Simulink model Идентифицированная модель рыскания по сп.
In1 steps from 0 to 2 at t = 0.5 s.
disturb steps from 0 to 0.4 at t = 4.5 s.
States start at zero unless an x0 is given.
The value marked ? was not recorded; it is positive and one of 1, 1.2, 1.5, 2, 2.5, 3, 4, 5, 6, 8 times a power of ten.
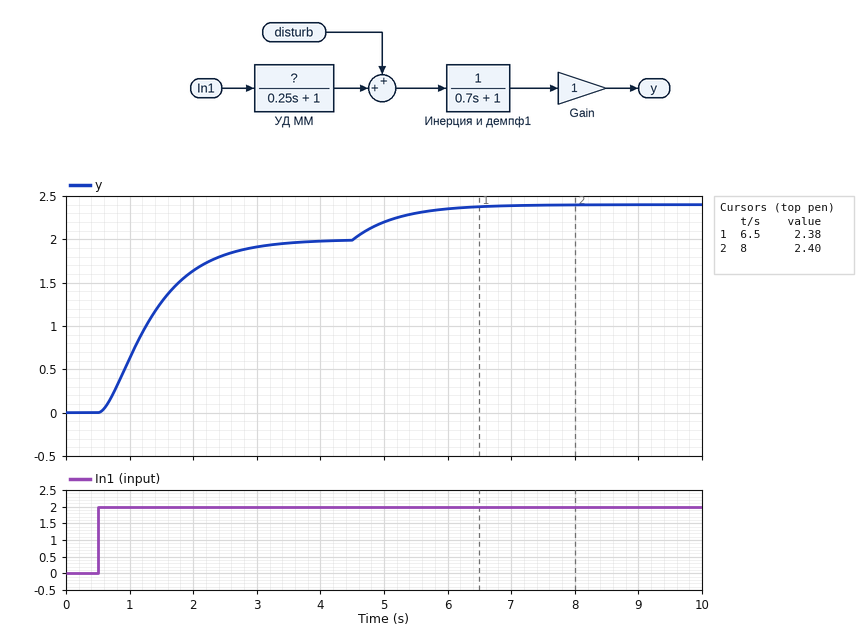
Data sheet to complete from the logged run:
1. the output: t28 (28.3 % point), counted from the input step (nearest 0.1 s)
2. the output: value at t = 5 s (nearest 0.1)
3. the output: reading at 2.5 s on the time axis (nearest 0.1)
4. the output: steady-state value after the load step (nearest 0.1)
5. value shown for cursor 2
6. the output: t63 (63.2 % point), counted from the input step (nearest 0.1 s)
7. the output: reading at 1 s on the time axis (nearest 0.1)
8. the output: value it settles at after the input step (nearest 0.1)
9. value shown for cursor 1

0.5 s
2.2
1.8
2.4
2.40
1.0 s
0.6
2.0
2.38
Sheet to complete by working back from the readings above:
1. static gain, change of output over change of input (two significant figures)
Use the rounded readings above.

1.0
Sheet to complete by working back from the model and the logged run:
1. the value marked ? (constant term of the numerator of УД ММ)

1
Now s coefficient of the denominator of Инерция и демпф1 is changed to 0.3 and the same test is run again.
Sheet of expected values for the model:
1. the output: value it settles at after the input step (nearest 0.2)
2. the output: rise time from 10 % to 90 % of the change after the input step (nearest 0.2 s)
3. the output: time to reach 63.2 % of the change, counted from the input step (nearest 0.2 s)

2.0
1.0 s
0.6 s
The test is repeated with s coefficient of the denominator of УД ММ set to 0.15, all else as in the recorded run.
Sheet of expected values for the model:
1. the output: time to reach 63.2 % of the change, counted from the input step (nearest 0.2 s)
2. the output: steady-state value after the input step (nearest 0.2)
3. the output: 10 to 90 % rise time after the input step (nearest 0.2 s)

0.8 s
2.0
1.6 s
